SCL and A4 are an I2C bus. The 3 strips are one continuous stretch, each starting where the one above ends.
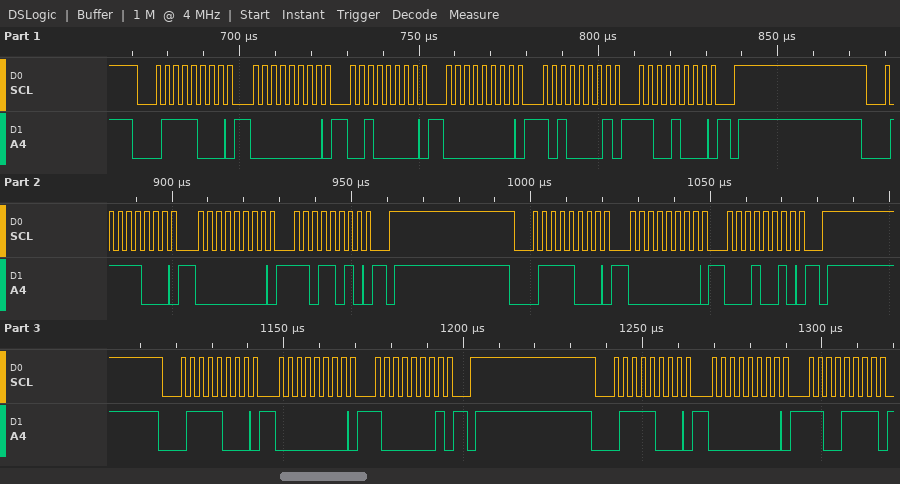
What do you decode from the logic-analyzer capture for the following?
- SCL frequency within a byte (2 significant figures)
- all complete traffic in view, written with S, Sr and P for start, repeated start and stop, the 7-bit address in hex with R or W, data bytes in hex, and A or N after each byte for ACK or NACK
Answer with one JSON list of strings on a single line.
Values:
["400 kHz", "S 3CW A 00 A 20 A 00 A A1 A C8 A P S 3CW A 00 A DA A P S 3CW A 00 A 12 A P S 3CW A 00 A 81 A P S 3CW A 00 A CF A"]
